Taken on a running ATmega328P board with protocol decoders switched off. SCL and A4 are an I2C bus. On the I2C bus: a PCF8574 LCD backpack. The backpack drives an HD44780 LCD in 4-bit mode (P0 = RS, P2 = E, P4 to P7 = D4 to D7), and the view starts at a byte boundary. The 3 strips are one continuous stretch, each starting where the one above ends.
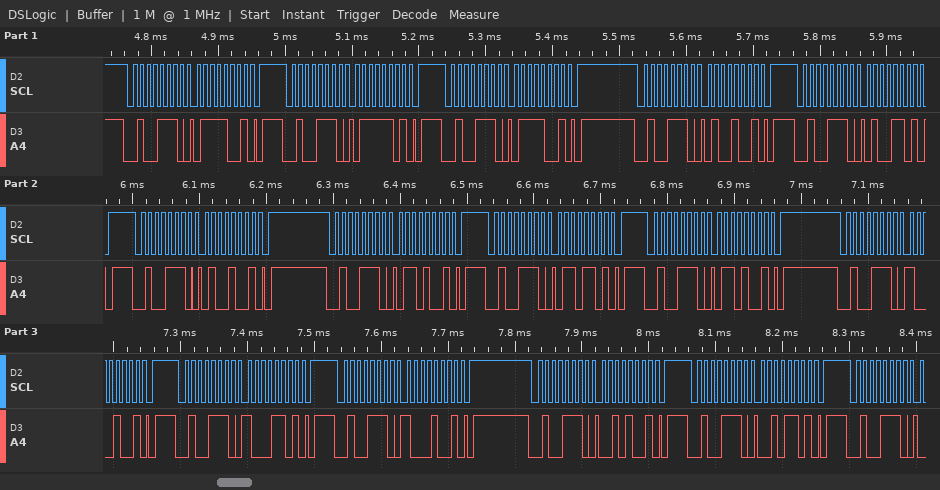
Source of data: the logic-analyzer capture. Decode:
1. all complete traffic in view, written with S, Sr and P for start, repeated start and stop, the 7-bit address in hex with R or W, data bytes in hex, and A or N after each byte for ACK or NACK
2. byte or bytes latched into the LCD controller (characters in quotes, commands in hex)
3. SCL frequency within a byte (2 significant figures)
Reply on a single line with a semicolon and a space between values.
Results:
S 27W A 79 A P S 27W A 7D A P S 27W A 79 A P S 27W A 49 A P S 27W A 4D A P S 27W A 49 A P S 27W A 69 A P S 27W A 6D A P S 27W A 69 A P S 27W A 89 A P S 27W A 8D A P S 27W A 89 A P S 27W A 29 A P S 27W A 2D A P S 27W A; 't' 'h'; 100 kHz
